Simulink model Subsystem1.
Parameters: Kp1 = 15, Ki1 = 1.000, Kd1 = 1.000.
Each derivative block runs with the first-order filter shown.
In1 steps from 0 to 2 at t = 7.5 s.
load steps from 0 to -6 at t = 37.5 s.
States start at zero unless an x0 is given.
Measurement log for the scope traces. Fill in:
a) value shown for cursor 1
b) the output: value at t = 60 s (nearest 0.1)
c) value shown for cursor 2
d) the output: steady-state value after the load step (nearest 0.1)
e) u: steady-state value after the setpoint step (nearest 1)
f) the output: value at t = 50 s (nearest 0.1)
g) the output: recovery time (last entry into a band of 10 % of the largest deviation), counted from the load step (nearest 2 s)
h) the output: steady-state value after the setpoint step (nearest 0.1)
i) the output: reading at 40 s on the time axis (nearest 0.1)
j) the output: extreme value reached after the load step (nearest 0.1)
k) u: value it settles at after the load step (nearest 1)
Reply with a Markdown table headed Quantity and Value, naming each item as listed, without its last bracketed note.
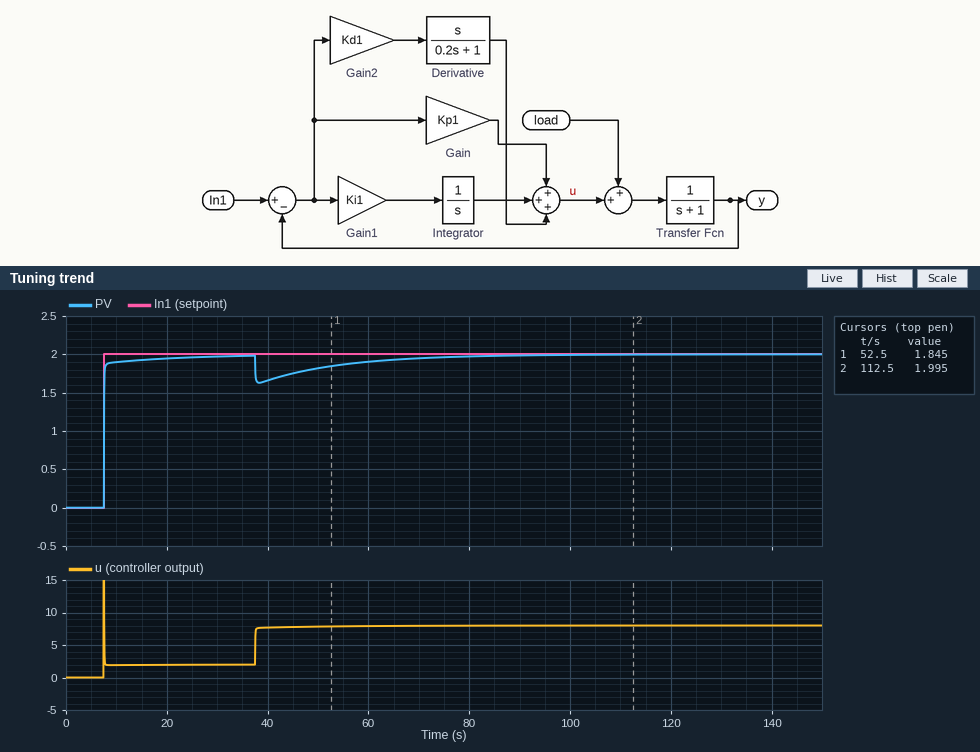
| Quantity | Value |
|---|---|
| value shown for cursor 1 | 1.845 |
| the output: value at t = 60 s | 1.9 |
| value shown for cursor 2 | 1.995 |
| the output: steady-state value after the load step | 2.0 |
| u: steady-state value after the setpoint step | 2 |
| the output: value at t = 50 s | 1.8 |
| the output: recovery time (last entry into a band of 10 % of the largest deviation), counted from the load step | 38 s |
| the output: steady-state value after the setpoint step | 2.0 |
| the output: reading at 40 s on the time axis | 1.7 |
| the output: extreme value reached after the load step | 1.6 |
| u: value it settles at after the load step | 8 |
